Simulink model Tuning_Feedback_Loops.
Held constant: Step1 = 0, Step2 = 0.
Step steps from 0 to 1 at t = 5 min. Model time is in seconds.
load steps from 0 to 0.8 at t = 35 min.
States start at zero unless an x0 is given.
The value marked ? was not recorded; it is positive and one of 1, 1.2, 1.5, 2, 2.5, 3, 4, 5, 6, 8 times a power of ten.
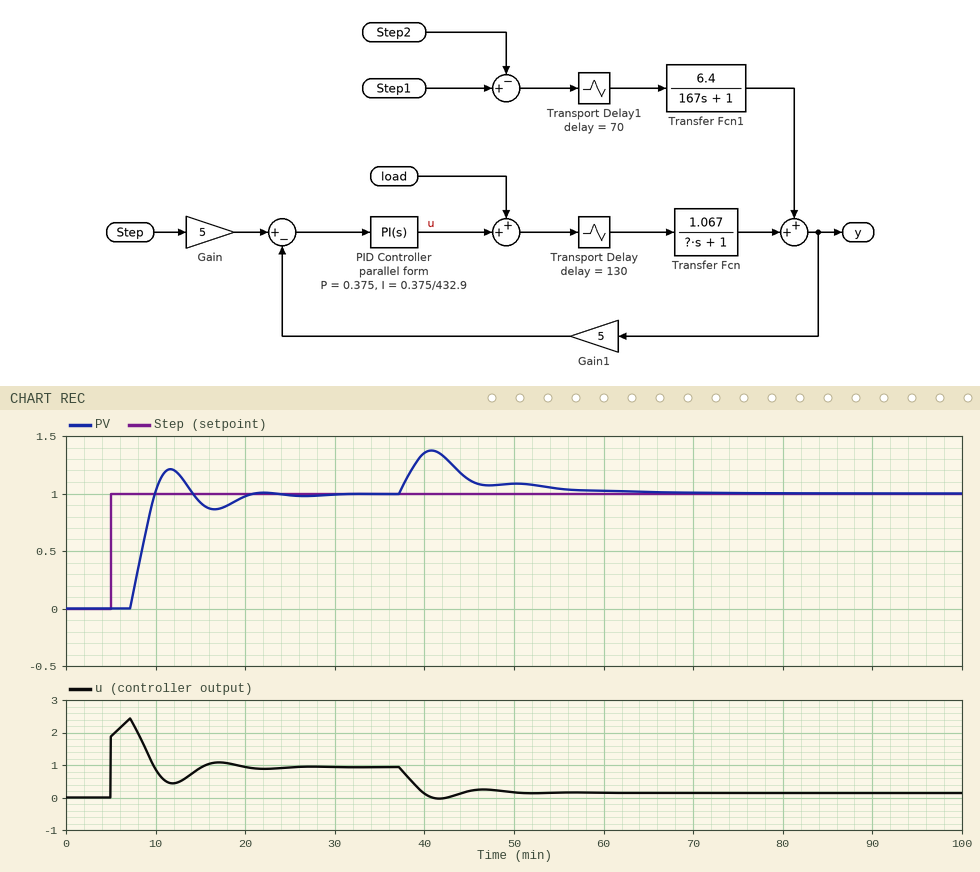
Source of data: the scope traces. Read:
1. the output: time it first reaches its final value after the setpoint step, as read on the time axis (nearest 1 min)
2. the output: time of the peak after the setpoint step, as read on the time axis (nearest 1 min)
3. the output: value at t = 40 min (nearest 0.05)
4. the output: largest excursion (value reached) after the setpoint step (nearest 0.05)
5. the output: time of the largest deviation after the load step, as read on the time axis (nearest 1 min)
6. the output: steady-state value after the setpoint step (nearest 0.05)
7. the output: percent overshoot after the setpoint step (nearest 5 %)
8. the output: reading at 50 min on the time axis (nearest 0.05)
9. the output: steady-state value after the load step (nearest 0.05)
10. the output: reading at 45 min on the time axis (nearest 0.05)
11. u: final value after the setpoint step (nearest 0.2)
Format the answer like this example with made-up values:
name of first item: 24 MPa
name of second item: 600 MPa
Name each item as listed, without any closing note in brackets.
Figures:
the output: time it first reaches its final value after the setpoint step, as read on the time axis: 10 min
the output: time of the peak after the setpoint step, as read on the time axis: 12 min
the output: value at t = 40 min: 1.35
the output: largest excursion (value reached) after the setpoint step: 1.20
the output: time of the largest deviation after the load step, as read on the time axis: 41 min
the output: steady-state value after the setpoint step: 1.00
the output: percent overshoot after the setpoint step: 20 %
the output: reading at 50 min on the time axis: 1.10
the output: steady-state value after the load step: 1.00
the output: reading at 45 min on the time axis: 1.10
u: final value after the setpoint step: 1.0
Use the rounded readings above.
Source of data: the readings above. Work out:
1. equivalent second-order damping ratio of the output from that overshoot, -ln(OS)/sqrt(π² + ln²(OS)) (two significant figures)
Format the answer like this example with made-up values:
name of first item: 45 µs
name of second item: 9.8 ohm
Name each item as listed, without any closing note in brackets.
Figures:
equivalent second-order damping ratio of the output from that overshoot, -ln(OS)/sqrt(π² + ln²(OS)): 0.46
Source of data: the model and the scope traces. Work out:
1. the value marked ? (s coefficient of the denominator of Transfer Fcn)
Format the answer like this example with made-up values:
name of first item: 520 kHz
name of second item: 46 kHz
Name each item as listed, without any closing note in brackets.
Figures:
the value marked ?: 300
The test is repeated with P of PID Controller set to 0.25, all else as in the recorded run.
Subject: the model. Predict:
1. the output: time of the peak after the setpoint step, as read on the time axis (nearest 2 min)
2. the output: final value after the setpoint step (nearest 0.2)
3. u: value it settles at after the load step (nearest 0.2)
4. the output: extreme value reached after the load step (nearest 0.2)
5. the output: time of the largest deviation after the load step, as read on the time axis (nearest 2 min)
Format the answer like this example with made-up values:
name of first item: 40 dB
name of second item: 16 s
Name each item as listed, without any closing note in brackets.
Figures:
the output: time of the peak after the setpoint step, as read on the time axis: 14 min
the output: final value after the setpoint step: 1.0
u: value it settles at after the load step: 0.2
the output: extreme value reached after the load step: 1.4
the output: time of the largest deviation after the load step, as read on the time axis: 42 min
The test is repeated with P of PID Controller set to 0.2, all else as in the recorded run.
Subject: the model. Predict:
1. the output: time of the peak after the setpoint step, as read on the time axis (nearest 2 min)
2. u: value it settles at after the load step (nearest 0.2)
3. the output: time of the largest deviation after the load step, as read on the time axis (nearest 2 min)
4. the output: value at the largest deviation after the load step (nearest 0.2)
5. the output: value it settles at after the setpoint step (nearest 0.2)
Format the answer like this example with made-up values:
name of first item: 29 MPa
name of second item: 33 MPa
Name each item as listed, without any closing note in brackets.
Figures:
the output: time of the peak after the setpoint step, as read on the time axis: 16 min
u: value it settles at after the load step: 0.2
the output: time of the largest deviation after the load step, as read on the time axis: 42 min
the output: value at the largest deviation after the load step: 1.4
the output: value it settles at after the setpoint step: 1.0
